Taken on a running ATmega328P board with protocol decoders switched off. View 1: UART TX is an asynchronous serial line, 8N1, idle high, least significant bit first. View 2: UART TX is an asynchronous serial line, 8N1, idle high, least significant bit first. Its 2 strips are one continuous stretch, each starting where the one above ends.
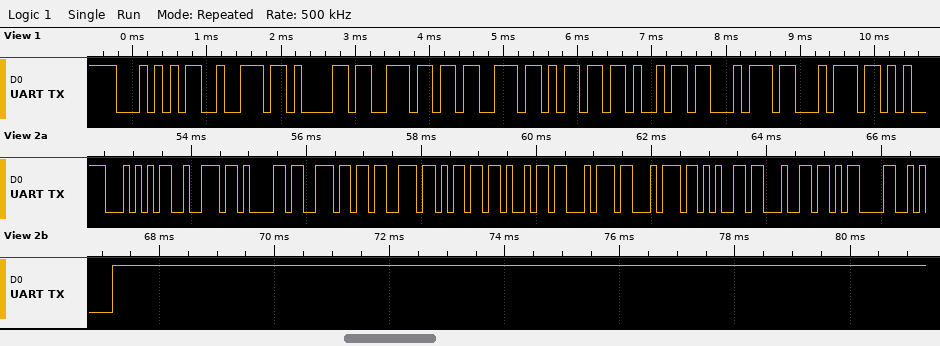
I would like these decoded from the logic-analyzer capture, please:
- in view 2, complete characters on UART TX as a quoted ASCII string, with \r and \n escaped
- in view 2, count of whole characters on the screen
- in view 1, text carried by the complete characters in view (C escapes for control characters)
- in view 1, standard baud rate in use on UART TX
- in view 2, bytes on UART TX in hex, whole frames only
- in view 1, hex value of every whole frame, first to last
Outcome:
"Transmitted\r\n"
13
"Transmitt"
9600 baud
54 72 61 6E 73 6D 69 74 74 65 64 0D 0A
54 72 61 6E 73 6D 69 74 74
